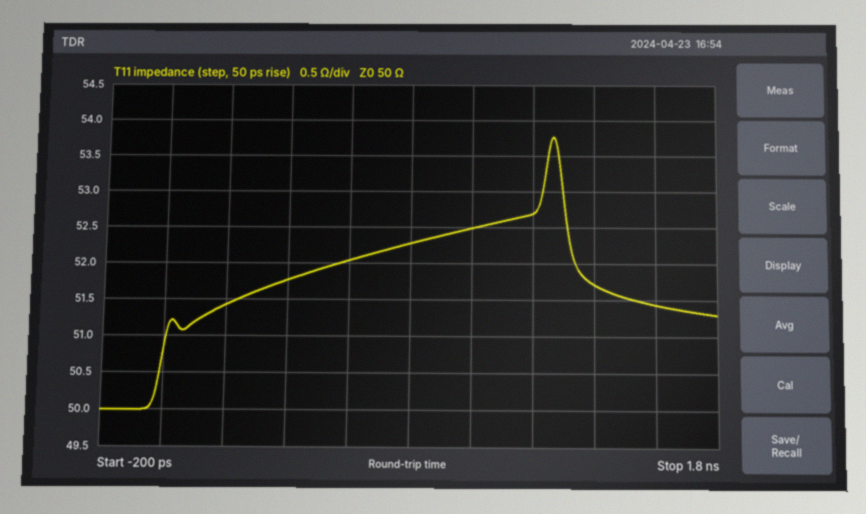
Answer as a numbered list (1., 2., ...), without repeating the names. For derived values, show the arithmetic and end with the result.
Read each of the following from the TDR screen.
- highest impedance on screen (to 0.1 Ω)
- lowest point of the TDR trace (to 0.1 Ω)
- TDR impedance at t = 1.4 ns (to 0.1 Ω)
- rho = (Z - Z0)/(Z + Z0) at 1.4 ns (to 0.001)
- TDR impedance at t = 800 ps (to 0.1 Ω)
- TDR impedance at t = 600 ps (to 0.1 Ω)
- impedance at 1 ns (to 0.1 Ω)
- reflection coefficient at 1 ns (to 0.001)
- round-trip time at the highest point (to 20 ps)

1. 53.8 Ω
2. 50.0 Ω
3. 51.7 Ω
4. (51.7 − 50)/(51.7 + 50) ≈ +0.017
5. 52.3 Ω
6. 52.0 Ω
7. 52.5 Ω
8. (52.5 − 50)/(52.5 + 50) ≈ +0.024
9. 1.26 ns
